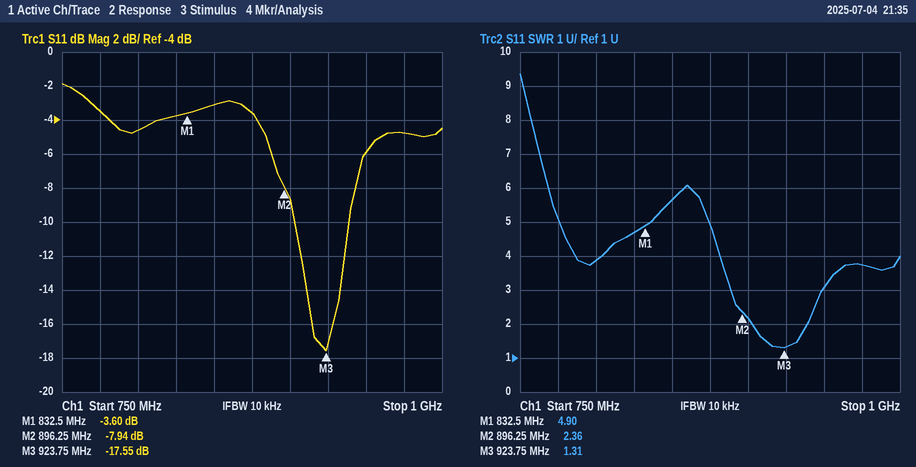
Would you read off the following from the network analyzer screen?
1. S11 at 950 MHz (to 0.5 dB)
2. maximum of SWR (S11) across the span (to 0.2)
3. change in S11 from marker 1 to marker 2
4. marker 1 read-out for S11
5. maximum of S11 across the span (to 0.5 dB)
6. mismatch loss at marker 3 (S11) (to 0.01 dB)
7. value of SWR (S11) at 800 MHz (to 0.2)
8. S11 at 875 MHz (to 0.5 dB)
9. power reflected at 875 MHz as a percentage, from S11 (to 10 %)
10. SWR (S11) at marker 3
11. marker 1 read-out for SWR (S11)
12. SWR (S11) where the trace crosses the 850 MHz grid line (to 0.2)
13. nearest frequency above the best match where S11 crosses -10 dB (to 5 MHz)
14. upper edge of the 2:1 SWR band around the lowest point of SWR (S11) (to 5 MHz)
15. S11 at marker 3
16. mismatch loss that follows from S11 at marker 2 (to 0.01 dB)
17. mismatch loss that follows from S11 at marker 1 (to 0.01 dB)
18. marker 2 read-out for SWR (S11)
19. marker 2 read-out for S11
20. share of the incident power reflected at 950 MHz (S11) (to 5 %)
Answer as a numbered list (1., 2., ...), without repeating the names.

1. -6.0 dB
2. 9.4
3. -4.34 dB
4. -3.60 dB
5. -2.0 dB
6. 0.08 dB
7. 3.8
8. -3.5 dB
9. 40 %
10. 1.31
11. 4.90
12. 5.6
13. 940 MHz
14. 940 MHz
15. -17.55 dB
16. 0.76 dB
17. 2.49 dB
18. 2.36
19. -7.94 dB
20. 25 %
